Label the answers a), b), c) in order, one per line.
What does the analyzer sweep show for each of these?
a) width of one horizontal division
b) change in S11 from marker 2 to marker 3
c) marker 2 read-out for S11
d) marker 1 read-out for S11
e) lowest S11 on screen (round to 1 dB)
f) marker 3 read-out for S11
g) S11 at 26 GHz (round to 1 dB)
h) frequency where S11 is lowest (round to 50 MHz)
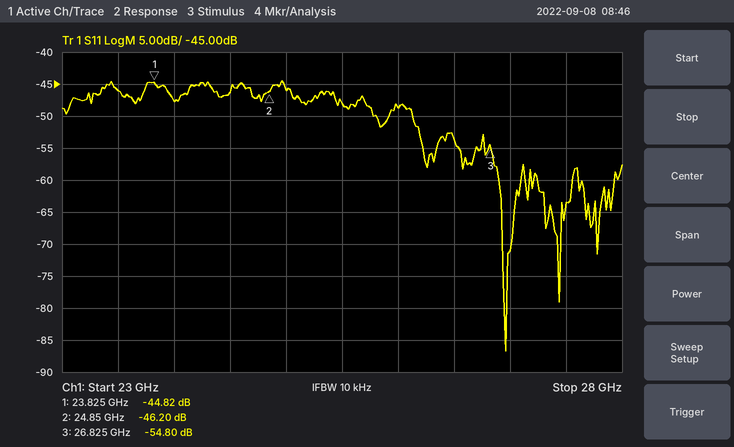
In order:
a) 500 MHz
b) -8.60 dB
c) -46.20 dB
d) -44.82 dB
e) -87 dB
f) -54.80 dB
g) -49 dB
h) 26.95 GHz
